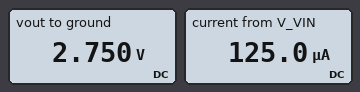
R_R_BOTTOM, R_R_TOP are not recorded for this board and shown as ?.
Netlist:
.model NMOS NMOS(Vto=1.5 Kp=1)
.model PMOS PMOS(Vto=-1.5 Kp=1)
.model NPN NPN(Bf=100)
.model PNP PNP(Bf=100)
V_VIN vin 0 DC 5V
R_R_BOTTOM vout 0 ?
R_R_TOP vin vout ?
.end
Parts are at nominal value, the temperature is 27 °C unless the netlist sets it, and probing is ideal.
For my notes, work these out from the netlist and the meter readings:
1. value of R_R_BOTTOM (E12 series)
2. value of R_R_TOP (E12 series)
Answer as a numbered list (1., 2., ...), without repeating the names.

1. 22 kΩ
2. 18 kΩ
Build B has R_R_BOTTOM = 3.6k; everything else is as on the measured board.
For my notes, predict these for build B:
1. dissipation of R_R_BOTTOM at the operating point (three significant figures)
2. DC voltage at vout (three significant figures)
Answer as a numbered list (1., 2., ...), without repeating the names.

1. 193 µW
2. 833 mV
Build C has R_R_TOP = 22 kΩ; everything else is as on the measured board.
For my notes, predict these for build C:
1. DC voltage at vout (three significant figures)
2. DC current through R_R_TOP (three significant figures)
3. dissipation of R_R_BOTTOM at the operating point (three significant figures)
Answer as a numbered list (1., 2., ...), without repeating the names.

1. 2.50 V
2. 114 µA
3. 284 µW
